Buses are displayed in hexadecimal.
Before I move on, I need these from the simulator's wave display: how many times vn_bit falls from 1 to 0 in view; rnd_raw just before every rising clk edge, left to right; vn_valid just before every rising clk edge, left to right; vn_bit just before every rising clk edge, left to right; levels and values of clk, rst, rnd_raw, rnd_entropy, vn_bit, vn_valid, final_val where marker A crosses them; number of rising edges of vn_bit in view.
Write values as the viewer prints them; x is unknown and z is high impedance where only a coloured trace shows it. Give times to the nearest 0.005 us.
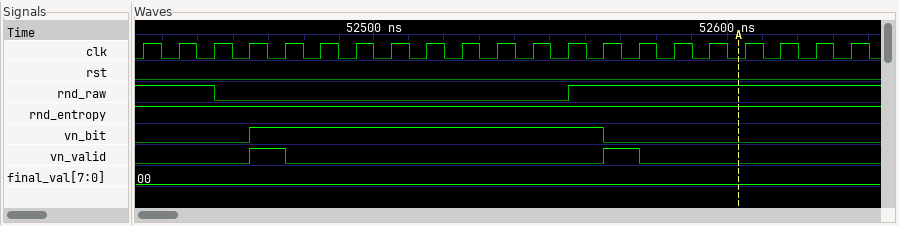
1
1 1 1 0 0 0 0 0 0 0 0 0 0 1 1 1 1 1 1 1 1
0 0 0 0 1 0 0 0 0 0 0 0 0 0 1 0 0 0 0 0 0
0 0 0 0 1 1 1 1 1 1 1 1 1 1 0 0 0 0 0 0 0
clk=0, rst=0, rnd_raw=1, rnd_entropy=1, vn_bit=0, vn_valid=0, final_val=00
1
